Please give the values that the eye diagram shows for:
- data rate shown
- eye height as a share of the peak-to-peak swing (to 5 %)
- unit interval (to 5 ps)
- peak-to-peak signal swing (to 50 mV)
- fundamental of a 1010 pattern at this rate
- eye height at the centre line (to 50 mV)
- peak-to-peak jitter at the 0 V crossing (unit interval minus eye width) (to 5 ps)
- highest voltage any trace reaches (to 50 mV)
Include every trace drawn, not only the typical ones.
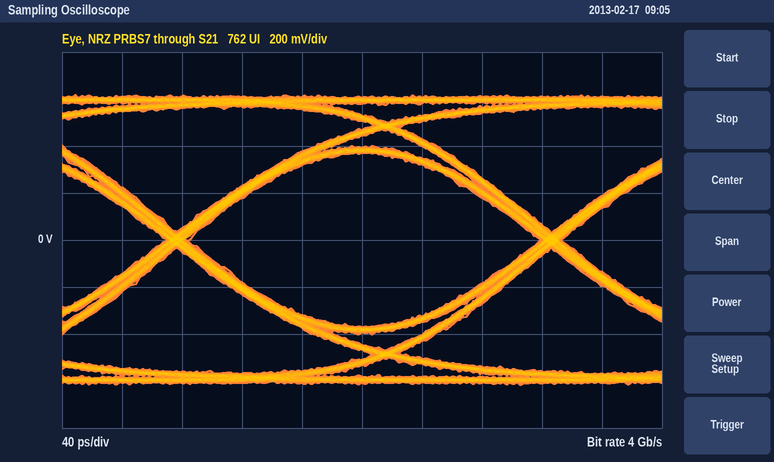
4 Gb/s
60 %
250 ps
1.25 V
2 GHz
750 mV
15 ps
600 mV
